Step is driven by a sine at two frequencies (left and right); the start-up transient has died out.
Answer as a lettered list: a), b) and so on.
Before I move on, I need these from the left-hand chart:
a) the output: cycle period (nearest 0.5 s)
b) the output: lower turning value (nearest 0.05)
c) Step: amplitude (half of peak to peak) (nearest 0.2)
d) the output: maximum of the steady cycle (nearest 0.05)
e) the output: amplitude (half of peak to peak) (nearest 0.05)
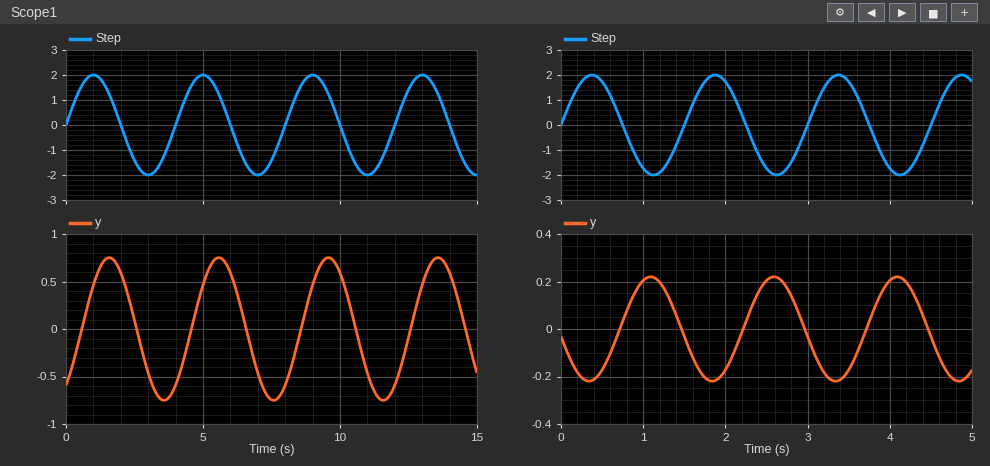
a) 4.0 s
b) -0.75
c) 2.0
d) 0.75
e) 0.75
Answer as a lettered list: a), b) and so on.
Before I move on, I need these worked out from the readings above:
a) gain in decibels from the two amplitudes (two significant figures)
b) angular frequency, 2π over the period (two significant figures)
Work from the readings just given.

a) -8.5 dB
b) 1.6 rad/s
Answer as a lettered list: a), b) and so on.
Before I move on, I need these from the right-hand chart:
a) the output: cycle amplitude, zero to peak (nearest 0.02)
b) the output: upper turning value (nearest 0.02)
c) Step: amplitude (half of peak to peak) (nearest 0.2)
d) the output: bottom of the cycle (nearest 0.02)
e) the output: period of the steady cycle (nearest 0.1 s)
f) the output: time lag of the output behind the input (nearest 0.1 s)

a) 0.22
b) 0.22
c) 2.0
d) -0.22
e) 1.5 s
f) 0.7 s
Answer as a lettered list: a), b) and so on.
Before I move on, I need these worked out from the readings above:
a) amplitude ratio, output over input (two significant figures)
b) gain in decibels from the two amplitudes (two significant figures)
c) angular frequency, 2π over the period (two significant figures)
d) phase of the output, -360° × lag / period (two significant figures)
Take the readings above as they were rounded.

a) 0.11
b) -19 dB
c) 4.2 rad/s
d) -170°
